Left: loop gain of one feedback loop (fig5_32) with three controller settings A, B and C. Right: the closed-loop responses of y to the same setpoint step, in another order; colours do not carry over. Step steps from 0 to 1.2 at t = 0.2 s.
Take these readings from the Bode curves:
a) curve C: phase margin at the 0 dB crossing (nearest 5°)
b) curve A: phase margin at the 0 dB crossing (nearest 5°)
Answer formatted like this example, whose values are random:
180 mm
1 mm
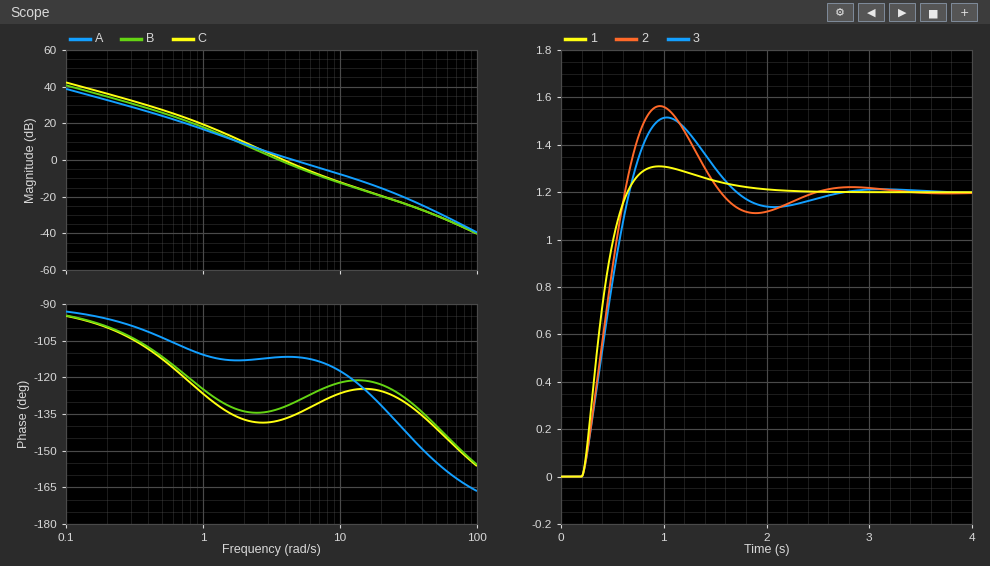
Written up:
45°
70°
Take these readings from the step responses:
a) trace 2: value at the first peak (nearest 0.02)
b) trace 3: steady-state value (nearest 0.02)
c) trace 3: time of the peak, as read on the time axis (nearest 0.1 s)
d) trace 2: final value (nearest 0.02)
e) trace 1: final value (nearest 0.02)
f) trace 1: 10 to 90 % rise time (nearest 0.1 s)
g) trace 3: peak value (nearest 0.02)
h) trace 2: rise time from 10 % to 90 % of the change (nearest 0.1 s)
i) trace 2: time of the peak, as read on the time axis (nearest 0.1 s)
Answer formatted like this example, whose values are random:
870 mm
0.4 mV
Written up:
1.56
1.20
1.0 s
1.20
1.20
0.3 s
1.52
0.3 s
1.0 s
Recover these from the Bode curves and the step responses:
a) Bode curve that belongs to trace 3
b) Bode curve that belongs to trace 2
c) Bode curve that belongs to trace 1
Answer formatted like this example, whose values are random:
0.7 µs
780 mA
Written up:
B
C
A
